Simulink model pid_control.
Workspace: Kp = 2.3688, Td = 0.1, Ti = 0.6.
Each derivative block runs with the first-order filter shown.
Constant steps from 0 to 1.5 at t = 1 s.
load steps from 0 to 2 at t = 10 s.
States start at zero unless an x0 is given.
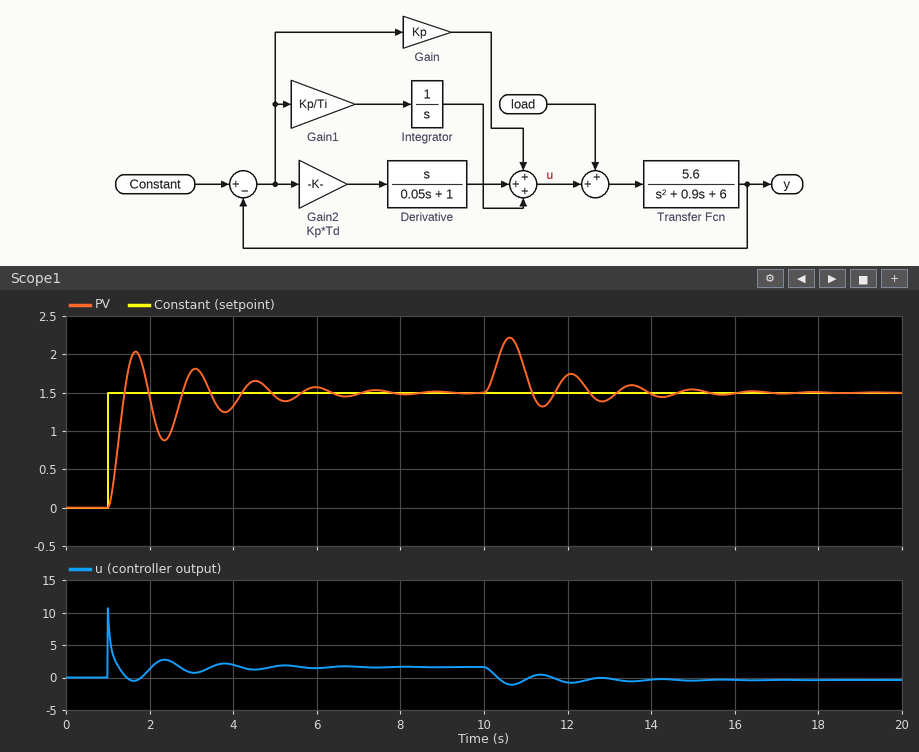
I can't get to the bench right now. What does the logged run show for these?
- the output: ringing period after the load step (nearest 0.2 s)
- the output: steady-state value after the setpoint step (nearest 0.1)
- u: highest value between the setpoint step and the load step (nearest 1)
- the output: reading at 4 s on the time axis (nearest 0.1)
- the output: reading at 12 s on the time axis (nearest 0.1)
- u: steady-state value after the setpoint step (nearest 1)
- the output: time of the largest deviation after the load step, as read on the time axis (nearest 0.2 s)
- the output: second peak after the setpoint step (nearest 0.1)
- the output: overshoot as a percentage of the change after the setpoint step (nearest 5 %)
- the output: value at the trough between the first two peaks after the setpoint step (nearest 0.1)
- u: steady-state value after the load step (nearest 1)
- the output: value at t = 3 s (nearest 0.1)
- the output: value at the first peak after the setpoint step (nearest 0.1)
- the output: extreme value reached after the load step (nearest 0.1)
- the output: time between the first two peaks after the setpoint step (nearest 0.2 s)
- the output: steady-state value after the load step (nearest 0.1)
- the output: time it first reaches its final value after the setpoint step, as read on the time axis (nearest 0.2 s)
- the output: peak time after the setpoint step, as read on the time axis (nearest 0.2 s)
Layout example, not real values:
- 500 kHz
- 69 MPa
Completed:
- 1.4 s
- 1.5
- 11
- 1.3
- 1.7
- 2
- 10.6 s
- 1.8
- 35 %
- 0.9
- 0
- 1.8
- 2.0
- 2.2
- 1.4 s
- 1.5
- 1.4 s
- 1.6 s
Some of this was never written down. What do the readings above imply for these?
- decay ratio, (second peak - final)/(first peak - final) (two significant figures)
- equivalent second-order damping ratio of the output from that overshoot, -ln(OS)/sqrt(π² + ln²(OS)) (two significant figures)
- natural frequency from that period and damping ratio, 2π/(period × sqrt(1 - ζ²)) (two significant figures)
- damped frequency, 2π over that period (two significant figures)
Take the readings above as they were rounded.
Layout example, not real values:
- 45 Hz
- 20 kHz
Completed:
- 0.60
- 0.32
- 4.7 rad/s
- 4.5 rad/s
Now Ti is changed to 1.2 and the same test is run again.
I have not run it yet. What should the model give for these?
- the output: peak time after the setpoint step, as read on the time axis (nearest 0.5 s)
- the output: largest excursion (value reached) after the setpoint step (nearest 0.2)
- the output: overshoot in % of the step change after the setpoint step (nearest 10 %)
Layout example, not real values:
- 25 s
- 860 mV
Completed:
- 1.5 s
- 1.8
- 20 %
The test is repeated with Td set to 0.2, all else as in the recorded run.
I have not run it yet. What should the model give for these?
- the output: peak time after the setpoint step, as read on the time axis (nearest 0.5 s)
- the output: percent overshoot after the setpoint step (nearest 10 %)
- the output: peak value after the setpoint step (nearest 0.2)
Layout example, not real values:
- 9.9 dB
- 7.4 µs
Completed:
- 1.5 s
- 20 %
- 1.8
